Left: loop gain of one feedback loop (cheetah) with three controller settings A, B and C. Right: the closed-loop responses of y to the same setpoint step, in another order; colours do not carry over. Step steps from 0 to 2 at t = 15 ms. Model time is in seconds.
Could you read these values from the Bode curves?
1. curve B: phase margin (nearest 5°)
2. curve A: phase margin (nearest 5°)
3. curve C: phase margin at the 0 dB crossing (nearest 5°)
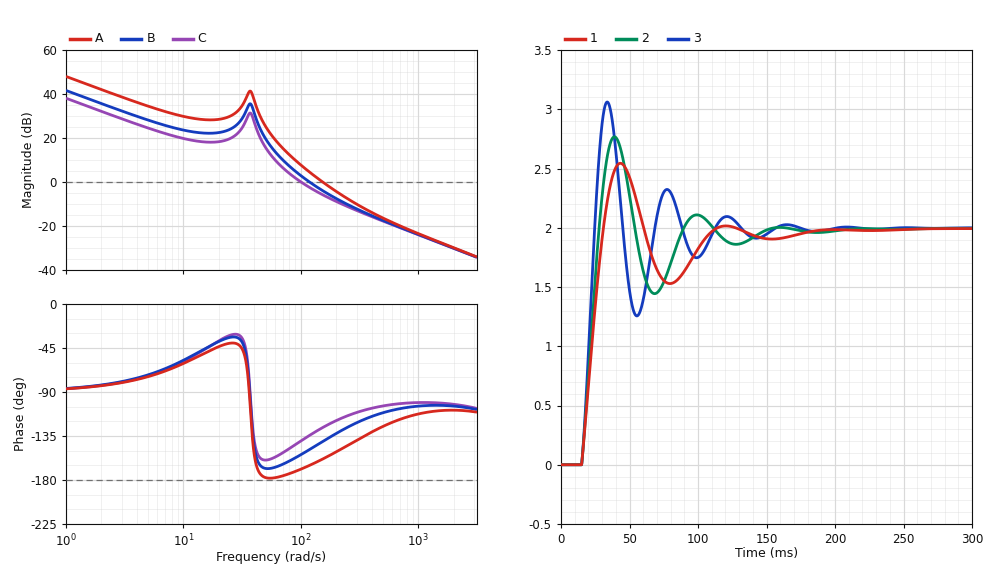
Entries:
30°
20°
40°
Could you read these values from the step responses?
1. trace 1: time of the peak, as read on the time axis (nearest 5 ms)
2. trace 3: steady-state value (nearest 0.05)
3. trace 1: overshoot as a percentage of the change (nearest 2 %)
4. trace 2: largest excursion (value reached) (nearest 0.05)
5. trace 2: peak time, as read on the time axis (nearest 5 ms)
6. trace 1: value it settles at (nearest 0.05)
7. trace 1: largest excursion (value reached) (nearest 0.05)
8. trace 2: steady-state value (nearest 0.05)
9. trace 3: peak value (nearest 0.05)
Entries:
45 ms
2.00
28 %
2.75
40 ms
2.00
2.55
2.00
3.05
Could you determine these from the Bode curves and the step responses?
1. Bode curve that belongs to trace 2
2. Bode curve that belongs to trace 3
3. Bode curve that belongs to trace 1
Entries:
B
A
C
